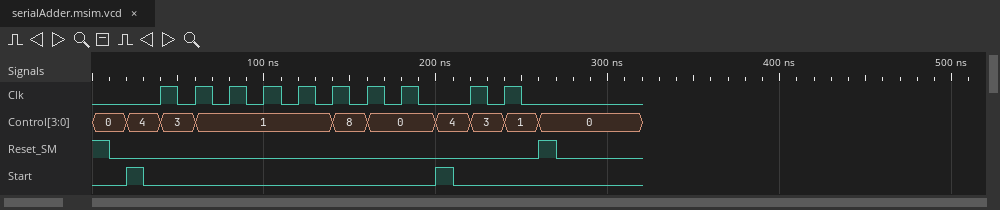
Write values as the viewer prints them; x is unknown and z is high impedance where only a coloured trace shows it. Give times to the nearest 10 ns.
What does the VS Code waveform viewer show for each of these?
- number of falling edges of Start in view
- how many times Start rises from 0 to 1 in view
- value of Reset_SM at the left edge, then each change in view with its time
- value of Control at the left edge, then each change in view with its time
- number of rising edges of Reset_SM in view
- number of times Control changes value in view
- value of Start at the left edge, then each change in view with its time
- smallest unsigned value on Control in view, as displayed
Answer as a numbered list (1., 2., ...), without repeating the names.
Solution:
1. 2
2. 2
3. 1, 0 at 10 ns, 1 at 260 ns, 0 at 270 ns
4. 0, 4 at 20 ns, 3 at 40 ns, 1 at 60 ns, 8 at 140 ns, 0 at 160 ns, 4 at 200 ns, 3 at 220 ns, 1 at 240 ns, 0 at 260 ns
5. 1
6. 9
7. 0, 1 at 20 ns, 0 at 30 ns, 1 at 200 ns, 0 at 210 ns
8. 0
